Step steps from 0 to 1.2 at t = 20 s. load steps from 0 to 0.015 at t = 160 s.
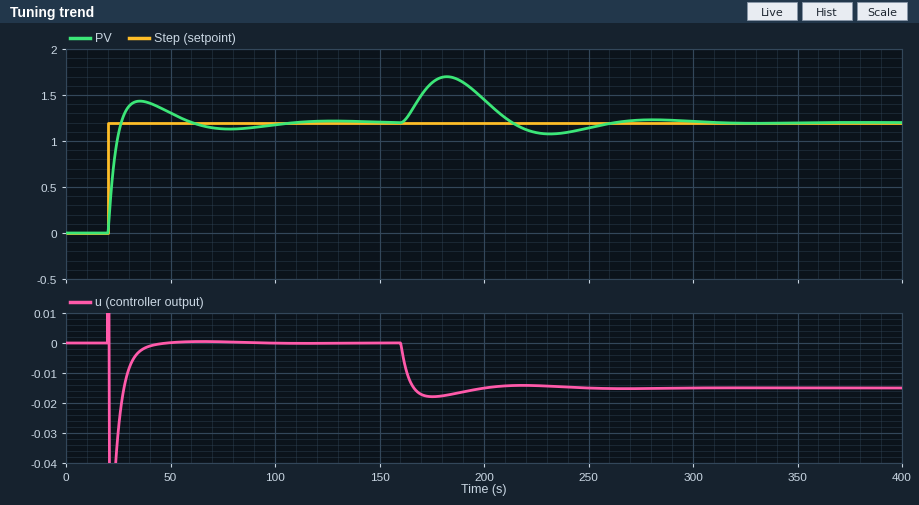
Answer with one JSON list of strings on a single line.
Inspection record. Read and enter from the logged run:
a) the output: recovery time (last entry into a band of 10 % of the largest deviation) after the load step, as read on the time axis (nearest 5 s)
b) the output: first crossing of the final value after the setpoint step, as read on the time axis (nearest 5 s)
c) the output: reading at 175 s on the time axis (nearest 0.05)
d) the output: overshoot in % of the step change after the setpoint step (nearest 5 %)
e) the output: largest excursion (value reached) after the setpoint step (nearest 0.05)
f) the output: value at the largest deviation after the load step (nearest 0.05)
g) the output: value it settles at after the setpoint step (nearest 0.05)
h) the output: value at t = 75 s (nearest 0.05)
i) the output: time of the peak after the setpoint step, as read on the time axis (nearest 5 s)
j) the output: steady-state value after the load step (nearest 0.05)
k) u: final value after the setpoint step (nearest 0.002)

["250 s", "25 s", "1.65", "20 %", "1.45", "1.70", "1.20", "1.15", "35 s", "1.20", "0.000"]
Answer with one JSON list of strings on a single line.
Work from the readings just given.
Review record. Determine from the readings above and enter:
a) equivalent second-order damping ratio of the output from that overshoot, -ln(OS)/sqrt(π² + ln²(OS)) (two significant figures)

["0.46"]
